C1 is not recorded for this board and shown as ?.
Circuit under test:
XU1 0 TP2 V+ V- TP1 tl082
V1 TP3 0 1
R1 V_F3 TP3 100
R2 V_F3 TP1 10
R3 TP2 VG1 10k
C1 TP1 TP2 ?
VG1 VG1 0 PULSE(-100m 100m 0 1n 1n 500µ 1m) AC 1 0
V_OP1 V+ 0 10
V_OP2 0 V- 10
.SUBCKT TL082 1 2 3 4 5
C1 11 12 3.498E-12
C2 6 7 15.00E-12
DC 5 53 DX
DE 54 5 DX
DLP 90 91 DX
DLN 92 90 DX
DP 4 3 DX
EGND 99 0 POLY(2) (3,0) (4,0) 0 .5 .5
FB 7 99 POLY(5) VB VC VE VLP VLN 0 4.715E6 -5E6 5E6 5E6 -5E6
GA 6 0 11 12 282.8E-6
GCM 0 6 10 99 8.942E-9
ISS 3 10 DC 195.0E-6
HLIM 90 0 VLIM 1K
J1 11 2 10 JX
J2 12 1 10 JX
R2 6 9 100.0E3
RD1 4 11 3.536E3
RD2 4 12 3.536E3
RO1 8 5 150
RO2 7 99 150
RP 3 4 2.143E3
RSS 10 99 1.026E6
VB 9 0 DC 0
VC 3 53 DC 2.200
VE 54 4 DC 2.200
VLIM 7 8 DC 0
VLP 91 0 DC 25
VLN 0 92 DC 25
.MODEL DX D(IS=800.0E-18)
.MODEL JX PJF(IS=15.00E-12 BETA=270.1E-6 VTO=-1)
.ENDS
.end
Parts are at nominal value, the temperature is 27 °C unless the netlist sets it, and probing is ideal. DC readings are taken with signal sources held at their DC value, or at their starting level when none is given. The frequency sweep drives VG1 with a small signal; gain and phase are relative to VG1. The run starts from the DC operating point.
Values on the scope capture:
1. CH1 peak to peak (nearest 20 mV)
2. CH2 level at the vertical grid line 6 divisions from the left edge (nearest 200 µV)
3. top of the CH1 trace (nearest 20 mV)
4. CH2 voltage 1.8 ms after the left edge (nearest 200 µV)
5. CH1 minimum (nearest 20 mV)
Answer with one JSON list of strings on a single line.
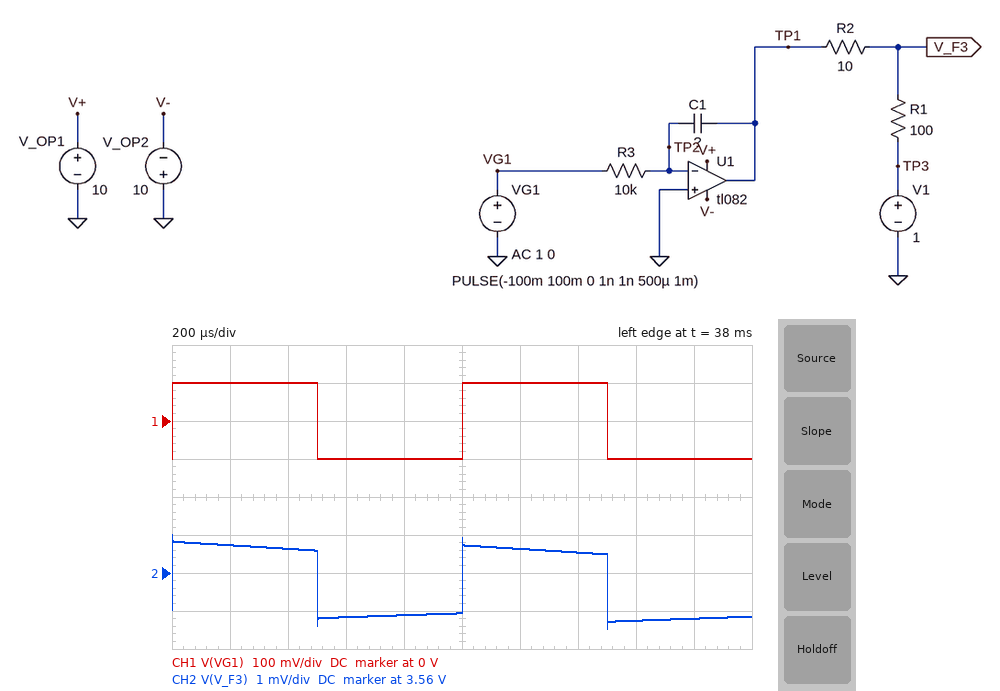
["200 mV", "3.5606 V", "100 mV", "3.5588 V", "-100 mV"]
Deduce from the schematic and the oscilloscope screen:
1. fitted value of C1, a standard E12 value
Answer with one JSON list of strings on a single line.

["2.7 µF"]
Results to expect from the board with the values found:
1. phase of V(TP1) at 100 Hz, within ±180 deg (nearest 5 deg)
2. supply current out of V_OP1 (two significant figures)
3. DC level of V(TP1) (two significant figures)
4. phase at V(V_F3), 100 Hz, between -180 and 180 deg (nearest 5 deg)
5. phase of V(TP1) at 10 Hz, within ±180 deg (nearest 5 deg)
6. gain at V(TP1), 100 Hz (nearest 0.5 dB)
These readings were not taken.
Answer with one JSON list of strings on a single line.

["10 deg", "9.5 mA", "3.8 V", "10 deg", "85 deg", "-39.5 dB"]
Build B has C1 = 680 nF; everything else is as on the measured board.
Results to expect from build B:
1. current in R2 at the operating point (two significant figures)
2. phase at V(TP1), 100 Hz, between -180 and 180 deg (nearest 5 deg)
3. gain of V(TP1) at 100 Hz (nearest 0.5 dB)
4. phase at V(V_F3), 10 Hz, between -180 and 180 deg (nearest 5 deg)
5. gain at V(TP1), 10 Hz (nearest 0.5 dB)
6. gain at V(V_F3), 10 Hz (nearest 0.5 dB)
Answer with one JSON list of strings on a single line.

["26 mA", "45 deg", "-38.5 dB", "145 deg", "-31.5 dB", "-32.5 dB"]
